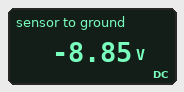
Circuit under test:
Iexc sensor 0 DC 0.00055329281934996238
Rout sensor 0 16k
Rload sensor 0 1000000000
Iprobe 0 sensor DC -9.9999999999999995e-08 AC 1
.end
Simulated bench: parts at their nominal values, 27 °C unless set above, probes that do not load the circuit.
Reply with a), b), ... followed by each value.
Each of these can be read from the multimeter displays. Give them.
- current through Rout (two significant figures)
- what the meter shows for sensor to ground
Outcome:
a) 550 µA
b) -8.85 V
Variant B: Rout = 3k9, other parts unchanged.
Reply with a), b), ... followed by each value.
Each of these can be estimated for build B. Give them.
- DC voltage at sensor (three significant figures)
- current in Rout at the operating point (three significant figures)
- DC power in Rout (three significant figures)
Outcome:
a) -2.16 V
b) 553 µA
c) 1.19 mW
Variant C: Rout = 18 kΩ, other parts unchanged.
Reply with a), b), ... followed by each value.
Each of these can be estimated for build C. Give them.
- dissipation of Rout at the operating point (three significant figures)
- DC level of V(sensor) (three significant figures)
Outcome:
a) 5.51 mW
b) -9.96 V
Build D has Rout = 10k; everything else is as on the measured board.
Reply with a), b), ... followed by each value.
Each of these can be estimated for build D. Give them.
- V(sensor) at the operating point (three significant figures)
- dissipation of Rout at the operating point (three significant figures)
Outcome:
a) -5.53 V
b) 3.06 mW
